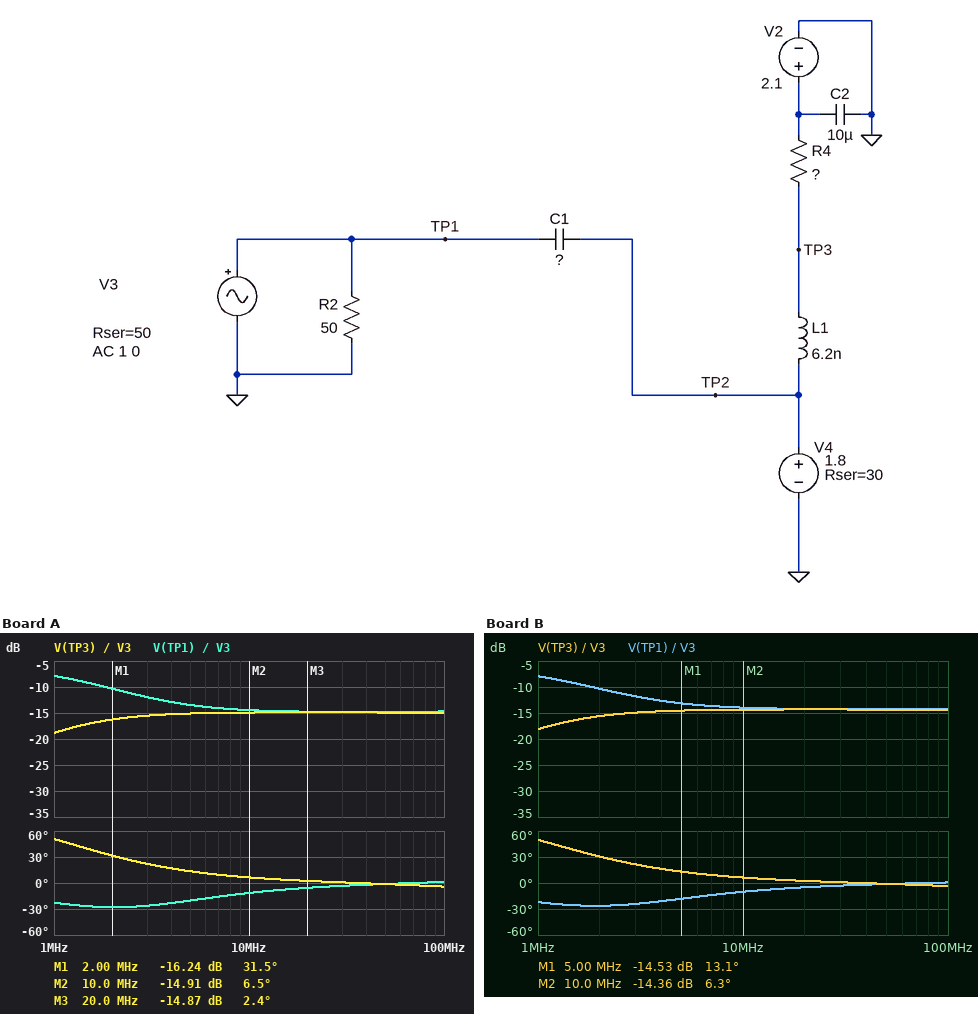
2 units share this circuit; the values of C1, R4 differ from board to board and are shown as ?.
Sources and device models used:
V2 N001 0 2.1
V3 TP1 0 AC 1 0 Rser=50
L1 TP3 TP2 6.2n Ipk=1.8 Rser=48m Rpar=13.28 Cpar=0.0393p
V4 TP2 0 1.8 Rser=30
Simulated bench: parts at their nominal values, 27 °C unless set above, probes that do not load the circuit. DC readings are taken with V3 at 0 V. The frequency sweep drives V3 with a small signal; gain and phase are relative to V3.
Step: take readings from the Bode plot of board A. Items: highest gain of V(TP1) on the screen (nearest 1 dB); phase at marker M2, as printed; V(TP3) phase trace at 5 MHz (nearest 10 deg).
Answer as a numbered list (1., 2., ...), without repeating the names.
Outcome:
1. -8 dB
2. 6.5 deg
3. 10 deg
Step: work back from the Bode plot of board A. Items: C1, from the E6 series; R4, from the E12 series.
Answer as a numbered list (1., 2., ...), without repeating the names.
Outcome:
1. 3.3 nF
2. 27 Ω
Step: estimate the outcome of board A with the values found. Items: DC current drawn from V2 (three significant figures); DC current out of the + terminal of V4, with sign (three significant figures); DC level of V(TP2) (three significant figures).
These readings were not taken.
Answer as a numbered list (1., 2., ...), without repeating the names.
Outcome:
1. 5.26 mA
2. -5.26 mA
3. 1.96 V
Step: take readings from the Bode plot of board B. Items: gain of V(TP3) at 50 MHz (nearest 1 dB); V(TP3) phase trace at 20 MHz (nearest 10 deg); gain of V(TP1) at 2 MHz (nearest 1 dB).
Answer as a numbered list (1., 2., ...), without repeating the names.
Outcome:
1. -14 dB
2. 0 deg
3. -10 dB
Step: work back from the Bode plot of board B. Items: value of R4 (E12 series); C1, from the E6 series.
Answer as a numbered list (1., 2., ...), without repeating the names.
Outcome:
1. 33 Ω
2. 3.3 nF
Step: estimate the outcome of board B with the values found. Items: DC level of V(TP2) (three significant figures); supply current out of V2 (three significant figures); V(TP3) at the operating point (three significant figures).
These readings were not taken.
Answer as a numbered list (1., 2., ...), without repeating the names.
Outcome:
1. 1.94 V
2. 4.76 mA
3. 1.94 V
